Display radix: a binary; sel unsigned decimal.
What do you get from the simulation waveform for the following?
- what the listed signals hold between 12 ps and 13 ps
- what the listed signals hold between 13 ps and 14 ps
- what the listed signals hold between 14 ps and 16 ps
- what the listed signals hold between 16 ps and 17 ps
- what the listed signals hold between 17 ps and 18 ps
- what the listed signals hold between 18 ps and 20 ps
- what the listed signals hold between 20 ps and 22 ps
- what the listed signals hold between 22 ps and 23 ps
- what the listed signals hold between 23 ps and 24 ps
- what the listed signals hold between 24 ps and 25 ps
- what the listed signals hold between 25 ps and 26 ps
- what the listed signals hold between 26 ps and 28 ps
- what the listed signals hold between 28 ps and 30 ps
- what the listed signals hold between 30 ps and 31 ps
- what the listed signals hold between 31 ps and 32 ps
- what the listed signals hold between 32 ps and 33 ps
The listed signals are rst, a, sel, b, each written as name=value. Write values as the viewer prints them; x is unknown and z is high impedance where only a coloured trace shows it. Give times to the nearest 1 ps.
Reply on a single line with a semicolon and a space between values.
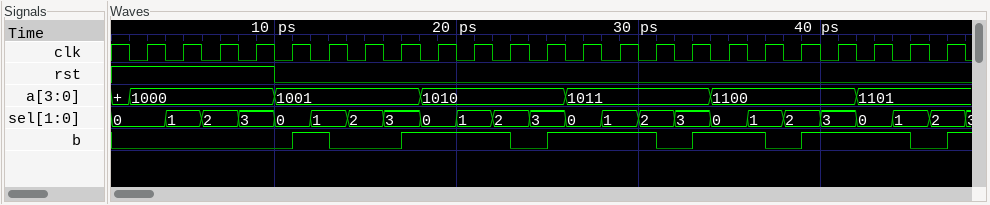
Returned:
rst=0, a=1001, sel=1, b=1; rst=0, a=1001, sel=1, b=0; rst=0, a=1001, sel=2, b=0; rst=0, a=1001, sel=3, b=0; rst=0, a=1001, sel=3, b=1; rst=0, a=1010, sel=0, b=1; rst=0, a=1010, sel=1, b=1; rst=0, a=1010, sel=2, b=1; rst=0, a=1010, sel=2, b=0; rst=0, a=1010, sel=3, b=0; rst=0, a=1010, sel=3, b=1; rst=0, a=1011, sel=0, b=1; rst=0, a=1011, sel=1, b=1; rst=0, a=1011, sel=2, b=1; rst=0, a=1011, sel=2, b=0; rst=0, a=1011, sel=3, b=0
